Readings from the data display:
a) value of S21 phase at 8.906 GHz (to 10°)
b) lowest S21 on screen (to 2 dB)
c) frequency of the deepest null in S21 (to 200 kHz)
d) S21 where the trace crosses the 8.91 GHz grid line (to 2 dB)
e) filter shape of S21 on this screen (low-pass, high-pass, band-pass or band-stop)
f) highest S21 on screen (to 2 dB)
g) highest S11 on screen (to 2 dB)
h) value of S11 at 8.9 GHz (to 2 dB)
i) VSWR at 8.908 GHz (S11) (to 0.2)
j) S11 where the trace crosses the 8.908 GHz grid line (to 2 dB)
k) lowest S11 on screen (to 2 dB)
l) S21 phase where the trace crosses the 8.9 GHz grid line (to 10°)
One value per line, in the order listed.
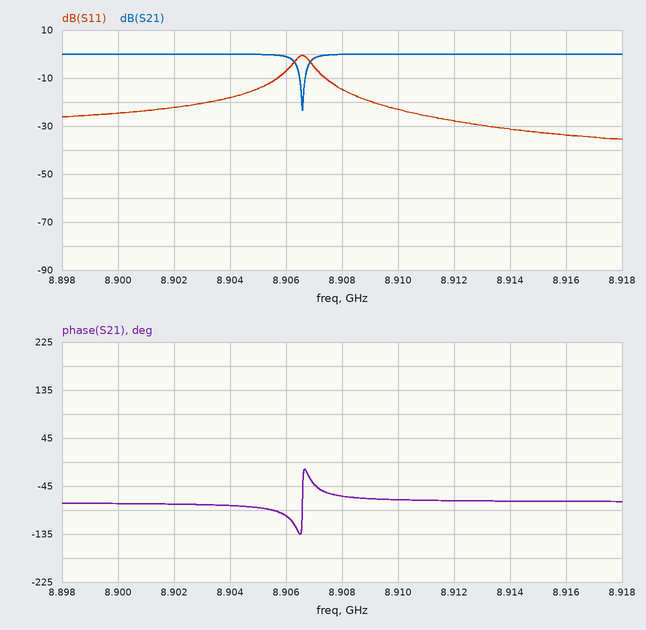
-100°
-24 dB
8.9066 GHz
0 dB
band-stop
0 dB
0 dB
-24 dB
1.4
-14 dB
-36 dB
-80°
